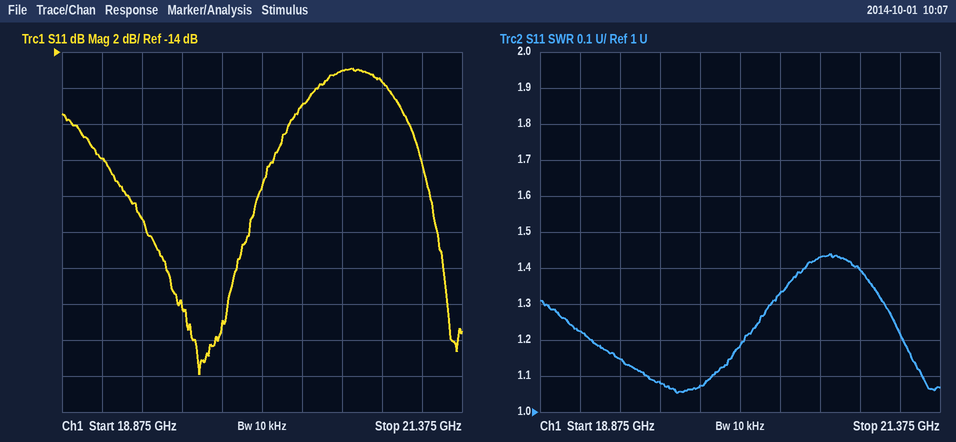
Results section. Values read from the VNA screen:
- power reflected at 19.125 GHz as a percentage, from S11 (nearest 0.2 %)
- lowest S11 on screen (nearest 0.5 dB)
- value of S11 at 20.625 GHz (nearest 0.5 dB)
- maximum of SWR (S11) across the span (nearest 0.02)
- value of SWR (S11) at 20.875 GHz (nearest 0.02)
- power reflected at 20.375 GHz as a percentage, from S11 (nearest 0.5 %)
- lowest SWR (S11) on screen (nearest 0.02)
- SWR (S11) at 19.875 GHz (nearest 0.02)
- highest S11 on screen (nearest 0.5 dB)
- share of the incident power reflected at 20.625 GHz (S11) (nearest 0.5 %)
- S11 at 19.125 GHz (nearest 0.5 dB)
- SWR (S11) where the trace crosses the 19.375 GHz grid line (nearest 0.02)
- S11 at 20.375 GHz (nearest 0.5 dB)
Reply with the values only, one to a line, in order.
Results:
1.0 %
-32.0 dB
-15.0 dB
1.44
1.40
2.0 %
1.06
1.08
-15.0 dB
3.0 %
-20.0 dB
1.14
-17.0 dB
